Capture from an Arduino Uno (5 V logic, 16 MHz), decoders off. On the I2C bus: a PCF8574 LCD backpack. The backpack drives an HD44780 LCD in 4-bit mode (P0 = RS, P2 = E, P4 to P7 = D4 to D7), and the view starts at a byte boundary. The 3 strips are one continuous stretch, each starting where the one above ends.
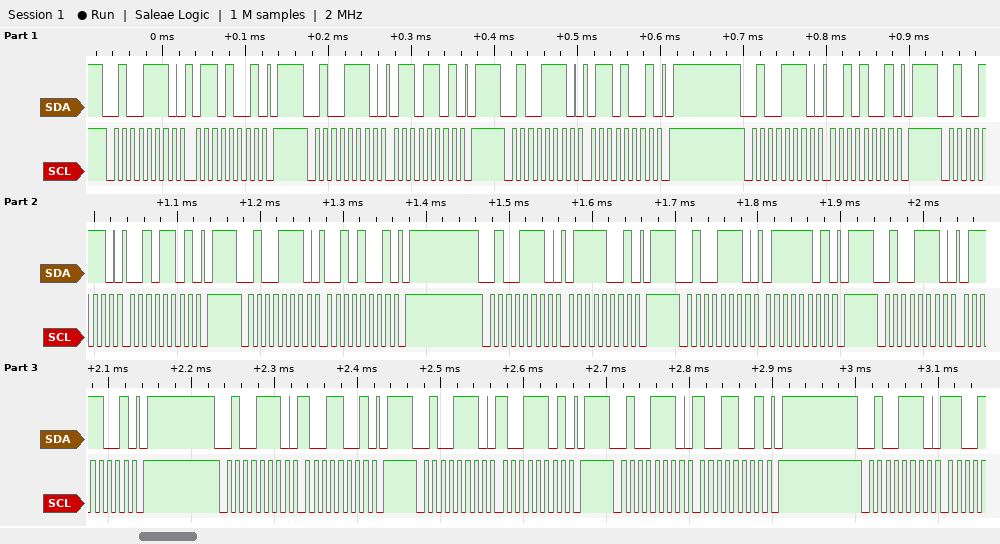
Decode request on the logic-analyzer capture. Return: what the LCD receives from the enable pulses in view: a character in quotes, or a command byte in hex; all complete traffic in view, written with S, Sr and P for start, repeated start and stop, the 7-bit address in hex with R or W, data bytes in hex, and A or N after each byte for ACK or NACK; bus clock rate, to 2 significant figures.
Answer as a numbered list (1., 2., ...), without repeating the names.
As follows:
1. 'b' 'y'
2. S 27W A 69 A P S 27W A 6D A P S 27W A 69 A P S 27W A 29 A P S 27W A 2D A P S 27W A 29 A P S 27W A 79 A P S 27W A 7D A P S 27W A 79 A P S 27W A 99 A P S 27W A 9D A P S 27W A 99 A P S 27W A
3. 100 kHz
